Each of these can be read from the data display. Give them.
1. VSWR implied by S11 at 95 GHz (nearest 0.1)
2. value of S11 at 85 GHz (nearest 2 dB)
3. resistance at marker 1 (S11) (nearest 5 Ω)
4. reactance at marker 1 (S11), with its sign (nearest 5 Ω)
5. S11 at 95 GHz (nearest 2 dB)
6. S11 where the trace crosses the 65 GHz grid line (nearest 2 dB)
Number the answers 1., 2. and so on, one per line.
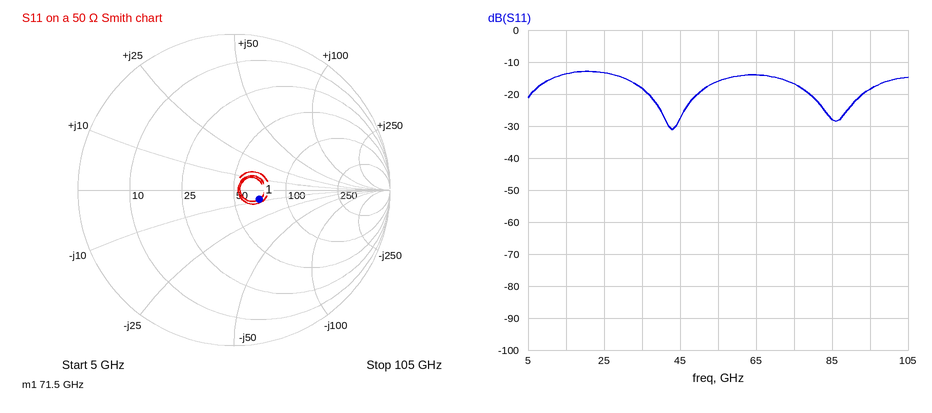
1. 1.3
2. -28 dB
3. 70 Ω
4. -10 Ω
5. -18 dB
6. -14 dB
